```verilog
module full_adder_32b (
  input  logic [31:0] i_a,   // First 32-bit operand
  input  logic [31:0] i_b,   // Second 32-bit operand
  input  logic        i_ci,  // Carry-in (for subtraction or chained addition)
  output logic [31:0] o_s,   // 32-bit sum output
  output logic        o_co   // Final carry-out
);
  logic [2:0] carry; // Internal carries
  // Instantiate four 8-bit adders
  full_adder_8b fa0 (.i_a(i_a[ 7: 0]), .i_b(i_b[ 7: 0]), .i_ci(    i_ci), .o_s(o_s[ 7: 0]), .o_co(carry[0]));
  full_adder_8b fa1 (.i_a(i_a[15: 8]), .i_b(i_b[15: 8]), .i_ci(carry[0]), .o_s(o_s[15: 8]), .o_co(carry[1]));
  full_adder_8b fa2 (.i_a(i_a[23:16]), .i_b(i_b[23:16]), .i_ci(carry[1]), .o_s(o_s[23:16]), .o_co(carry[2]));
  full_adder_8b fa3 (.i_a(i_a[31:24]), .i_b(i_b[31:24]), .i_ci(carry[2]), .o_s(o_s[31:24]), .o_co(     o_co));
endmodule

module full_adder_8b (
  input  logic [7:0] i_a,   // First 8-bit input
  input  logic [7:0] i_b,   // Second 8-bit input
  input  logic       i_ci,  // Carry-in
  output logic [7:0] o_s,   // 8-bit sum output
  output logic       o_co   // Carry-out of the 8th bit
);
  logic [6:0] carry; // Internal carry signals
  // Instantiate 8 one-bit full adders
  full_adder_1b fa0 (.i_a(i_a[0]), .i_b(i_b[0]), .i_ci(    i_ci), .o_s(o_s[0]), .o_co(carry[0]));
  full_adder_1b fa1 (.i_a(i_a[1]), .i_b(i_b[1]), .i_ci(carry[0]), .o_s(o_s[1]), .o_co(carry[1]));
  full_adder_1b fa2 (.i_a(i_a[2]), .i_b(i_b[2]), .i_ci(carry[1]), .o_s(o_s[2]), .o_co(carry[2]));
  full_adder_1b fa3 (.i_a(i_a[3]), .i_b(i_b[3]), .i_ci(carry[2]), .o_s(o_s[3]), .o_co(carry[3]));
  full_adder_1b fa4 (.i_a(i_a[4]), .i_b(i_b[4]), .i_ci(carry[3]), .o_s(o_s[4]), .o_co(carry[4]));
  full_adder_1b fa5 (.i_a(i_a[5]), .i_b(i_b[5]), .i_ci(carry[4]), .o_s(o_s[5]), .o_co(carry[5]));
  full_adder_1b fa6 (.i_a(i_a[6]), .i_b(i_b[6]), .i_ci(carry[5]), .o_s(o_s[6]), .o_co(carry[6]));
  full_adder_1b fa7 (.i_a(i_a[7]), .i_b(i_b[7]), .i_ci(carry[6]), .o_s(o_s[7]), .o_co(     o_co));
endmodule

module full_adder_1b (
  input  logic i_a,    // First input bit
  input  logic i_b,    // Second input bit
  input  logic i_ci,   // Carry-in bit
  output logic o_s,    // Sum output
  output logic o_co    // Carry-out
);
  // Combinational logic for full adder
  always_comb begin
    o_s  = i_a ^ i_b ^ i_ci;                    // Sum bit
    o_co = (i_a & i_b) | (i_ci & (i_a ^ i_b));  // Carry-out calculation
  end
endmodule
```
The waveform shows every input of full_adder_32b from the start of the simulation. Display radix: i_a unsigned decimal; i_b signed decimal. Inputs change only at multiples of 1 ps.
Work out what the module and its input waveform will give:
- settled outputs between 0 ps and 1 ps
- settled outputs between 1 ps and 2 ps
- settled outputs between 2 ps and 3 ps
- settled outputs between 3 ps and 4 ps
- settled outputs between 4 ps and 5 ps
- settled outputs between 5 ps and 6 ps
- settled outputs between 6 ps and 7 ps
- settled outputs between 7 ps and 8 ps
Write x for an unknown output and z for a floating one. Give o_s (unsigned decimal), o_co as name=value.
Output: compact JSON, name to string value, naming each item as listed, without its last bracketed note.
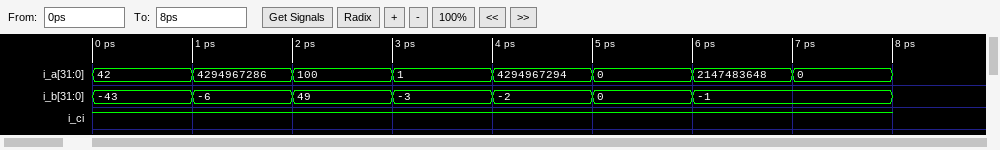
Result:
{"settled outputs between 0 ps and 1 ps": "o_s=0, o_co=1", "settled outputs between 1 ps and 2 ps": "o_s=4294967281, o_co=1", "settled outputs between 2 ps and 3 ps": "o_s=150, o_co=0", "settled outputs between 3 ps and 4 ps": "o_s=4294967295, o_co=0", "settled outputs between 4 ps and 5 ps": "o_s=4294967293, o_co=1", "settled outputs between 5 ps and 6 ps": "o_s=1, o_co=0", "settled outputs between 6 ps and 7 ps": "o_s=2147483648, o_co=1", "settled outputs between 7 ps and 8 ps": "o_s=0, o_co=1"}
